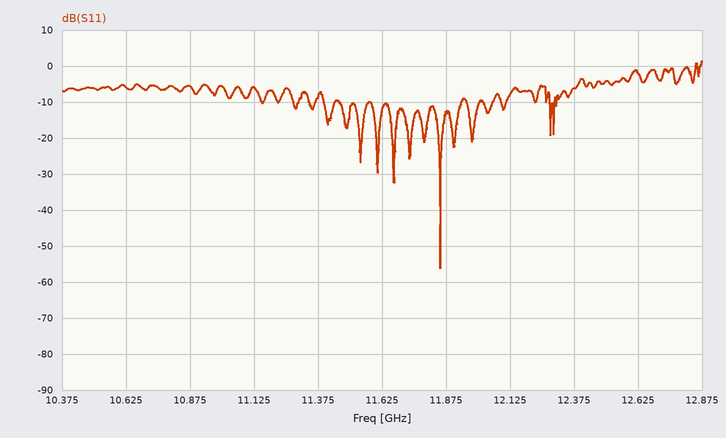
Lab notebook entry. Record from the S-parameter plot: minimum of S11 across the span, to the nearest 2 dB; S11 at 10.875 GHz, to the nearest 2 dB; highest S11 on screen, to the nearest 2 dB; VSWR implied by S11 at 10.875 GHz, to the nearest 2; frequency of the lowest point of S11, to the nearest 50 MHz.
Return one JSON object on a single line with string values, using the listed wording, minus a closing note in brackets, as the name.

{"minimum of S11 across the span, to the nearest 2 dB": "-56 dB", "S11 at 10.875 GHz, to the nearest 2 dB": "-6 dB", "highest S11 on screen, to the nearest 2 dB": "2 dB", "VSWR implied by S11 at 10.875 GHz, to the nearest 2": "4", "frequency of the lowest point of S11, to the nearest 50 MHz": "11.85 GHz"}
